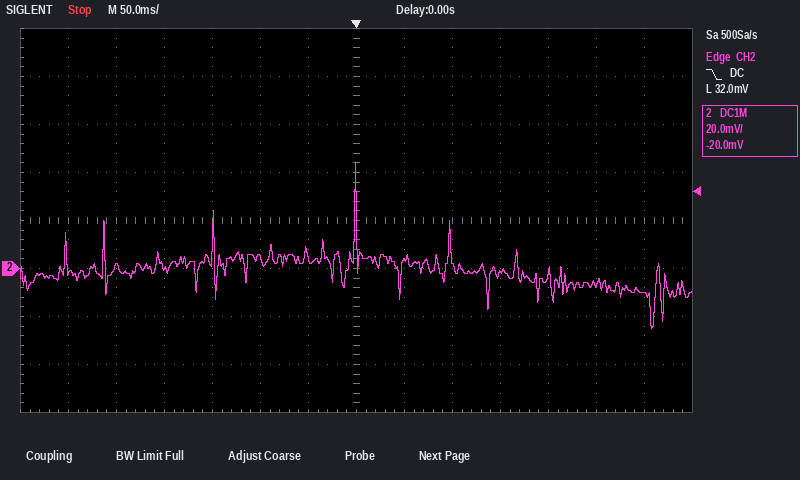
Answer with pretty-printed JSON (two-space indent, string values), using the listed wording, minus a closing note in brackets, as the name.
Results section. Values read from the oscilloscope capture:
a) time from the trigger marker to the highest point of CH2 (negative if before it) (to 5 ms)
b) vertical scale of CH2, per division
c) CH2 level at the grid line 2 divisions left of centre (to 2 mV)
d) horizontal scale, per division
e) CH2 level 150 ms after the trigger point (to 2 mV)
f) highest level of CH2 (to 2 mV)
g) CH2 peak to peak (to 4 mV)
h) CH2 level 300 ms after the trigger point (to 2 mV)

{
  "time from the trigger marker to the highest point of CH2 (negative if before it)": "0 ms",
  "vertical scale of CH2, per division": "20 mV",
  "CH2 level at the grid line 2 divisions left of centre": "4 mV",
  "horizontal scale, per division": "50 ms",
  "CH2 level 150 ms after the trigger point": "-2 mV",
  "highest level of CH2": "44 mV",
  "CH2 peak to peak": "68 mV",
  "CH2 level 300 ms after the trigger point": "-10 mV"
}
